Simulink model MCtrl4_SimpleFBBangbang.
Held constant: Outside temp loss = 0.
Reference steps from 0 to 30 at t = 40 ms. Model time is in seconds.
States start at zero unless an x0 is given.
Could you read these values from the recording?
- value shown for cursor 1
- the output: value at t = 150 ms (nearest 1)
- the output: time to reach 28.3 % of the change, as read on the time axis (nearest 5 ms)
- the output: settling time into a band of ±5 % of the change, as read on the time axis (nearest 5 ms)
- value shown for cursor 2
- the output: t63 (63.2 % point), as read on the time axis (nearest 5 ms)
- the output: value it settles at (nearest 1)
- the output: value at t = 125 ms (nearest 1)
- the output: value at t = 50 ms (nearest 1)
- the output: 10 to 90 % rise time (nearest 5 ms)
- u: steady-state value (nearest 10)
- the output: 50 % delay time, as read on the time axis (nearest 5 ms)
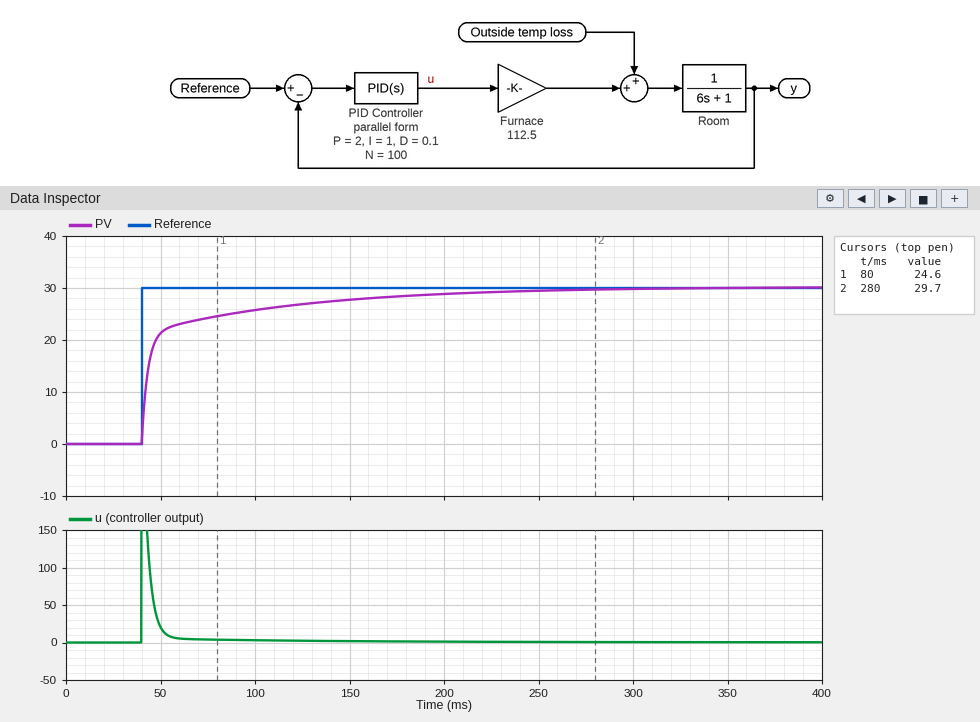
24.6
28
40 ms
185 ms
29.7
45 ms
30
27
21
90 ms
0
45 ms
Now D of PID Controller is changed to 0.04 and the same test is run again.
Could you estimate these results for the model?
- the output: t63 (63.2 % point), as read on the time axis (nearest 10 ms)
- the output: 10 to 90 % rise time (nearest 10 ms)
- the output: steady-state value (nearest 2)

60 ms
80 ms
30
